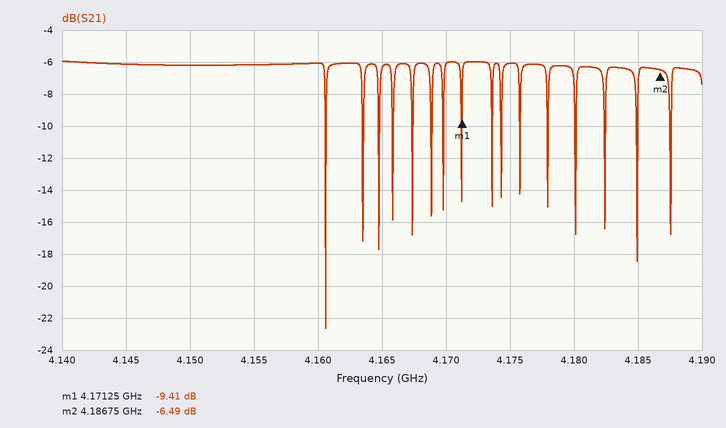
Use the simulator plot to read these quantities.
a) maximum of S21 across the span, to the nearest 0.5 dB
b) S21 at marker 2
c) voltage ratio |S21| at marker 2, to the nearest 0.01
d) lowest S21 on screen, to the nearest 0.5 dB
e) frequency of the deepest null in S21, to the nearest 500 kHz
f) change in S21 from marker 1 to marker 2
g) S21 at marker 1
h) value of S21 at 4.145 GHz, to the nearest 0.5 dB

-6.0 dB
-6.49 dB
0.47
-22.5 dB
4.1605 GHz
2.92 dB
-9.41 dB
-6.0 dB
